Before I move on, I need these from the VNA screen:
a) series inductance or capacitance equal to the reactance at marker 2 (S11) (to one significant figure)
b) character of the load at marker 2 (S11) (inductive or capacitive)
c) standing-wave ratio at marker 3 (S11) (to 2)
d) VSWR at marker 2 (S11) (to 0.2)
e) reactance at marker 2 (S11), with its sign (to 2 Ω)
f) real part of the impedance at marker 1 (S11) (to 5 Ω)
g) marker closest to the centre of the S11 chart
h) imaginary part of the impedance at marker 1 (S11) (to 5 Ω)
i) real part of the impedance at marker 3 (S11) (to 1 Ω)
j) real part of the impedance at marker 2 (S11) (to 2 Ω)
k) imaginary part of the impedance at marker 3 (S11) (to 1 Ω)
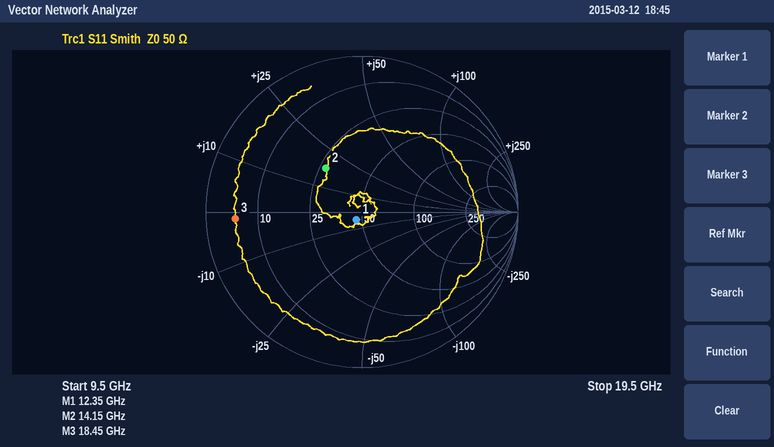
200 pH
inductive
10
2.2
+18 Ω
45 Ω
marker 1
-5 Ω
5 Ω
28 Ω
-1 Ω
